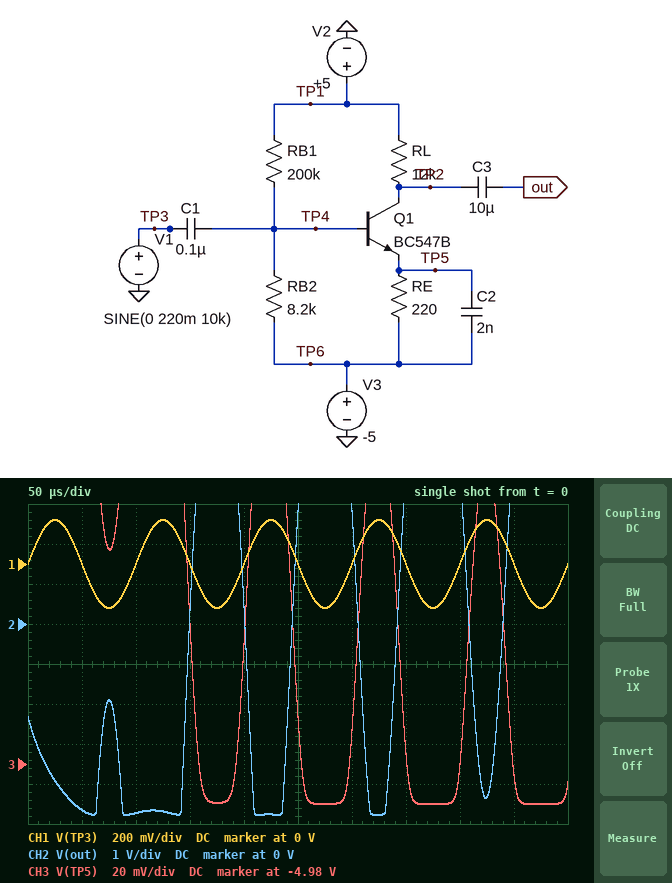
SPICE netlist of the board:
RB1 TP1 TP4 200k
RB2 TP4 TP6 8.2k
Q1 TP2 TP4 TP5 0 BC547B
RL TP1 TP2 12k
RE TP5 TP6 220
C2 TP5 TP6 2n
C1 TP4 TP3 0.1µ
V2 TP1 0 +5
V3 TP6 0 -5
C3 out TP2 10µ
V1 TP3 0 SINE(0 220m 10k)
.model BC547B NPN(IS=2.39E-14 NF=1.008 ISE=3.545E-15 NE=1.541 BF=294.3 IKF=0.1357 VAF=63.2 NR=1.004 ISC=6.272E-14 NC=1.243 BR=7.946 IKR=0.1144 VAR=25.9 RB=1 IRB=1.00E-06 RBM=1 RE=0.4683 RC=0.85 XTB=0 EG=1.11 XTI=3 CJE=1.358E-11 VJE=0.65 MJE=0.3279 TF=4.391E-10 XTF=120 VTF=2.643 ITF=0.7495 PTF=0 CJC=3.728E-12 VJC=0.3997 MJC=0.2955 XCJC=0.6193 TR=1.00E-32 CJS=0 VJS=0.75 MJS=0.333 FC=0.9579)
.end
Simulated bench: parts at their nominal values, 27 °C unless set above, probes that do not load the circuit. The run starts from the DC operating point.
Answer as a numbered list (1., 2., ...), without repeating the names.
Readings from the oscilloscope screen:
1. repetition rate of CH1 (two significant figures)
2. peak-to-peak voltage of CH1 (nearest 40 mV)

1. 10 kHz
2. 440 mV
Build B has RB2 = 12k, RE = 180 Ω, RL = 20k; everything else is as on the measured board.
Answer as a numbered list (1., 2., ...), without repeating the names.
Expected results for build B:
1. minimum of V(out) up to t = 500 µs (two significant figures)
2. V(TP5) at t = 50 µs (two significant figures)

1. -4.9 V
2. -4.8 V
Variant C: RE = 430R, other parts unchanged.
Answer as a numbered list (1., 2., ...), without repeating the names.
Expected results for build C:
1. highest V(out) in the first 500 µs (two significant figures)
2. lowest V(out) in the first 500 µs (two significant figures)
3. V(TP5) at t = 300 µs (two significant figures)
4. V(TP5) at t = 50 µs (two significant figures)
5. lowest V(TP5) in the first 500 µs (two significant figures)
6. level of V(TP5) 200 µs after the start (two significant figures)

1. 4.9 V
2. -4.6 V
3. -4.8 V
4. -3.9 V
5. -5.0 V
6. -4.7 V
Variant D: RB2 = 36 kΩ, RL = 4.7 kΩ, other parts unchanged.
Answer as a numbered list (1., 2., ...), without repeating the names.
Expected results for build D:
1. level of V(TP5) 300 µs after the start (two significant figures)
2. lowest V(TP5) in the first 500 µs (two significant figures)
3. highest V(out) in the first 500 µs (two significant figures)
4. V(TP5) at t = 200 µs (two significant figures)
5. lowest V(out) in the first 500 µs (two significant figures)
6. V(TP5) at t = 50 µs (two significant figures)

1. -4.7 V
2. -4.9 V
3. 3.0 V
4. -4.6 V
5. -4.5 V
6. -4.4 V
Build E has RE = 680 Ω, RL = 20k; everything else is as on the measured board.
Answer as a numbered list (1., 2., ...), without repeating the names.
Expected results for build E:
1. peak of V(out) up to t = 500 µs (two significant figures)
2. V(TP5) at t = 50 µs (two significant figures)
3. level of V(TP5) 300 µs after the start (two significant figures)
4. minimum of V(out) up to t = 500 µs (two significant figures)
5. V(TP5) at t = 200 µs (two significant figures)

1. 4.6 V
2. -3.3 V
3. -4.7 V
4. -4.6 V
5. -4.5 V
